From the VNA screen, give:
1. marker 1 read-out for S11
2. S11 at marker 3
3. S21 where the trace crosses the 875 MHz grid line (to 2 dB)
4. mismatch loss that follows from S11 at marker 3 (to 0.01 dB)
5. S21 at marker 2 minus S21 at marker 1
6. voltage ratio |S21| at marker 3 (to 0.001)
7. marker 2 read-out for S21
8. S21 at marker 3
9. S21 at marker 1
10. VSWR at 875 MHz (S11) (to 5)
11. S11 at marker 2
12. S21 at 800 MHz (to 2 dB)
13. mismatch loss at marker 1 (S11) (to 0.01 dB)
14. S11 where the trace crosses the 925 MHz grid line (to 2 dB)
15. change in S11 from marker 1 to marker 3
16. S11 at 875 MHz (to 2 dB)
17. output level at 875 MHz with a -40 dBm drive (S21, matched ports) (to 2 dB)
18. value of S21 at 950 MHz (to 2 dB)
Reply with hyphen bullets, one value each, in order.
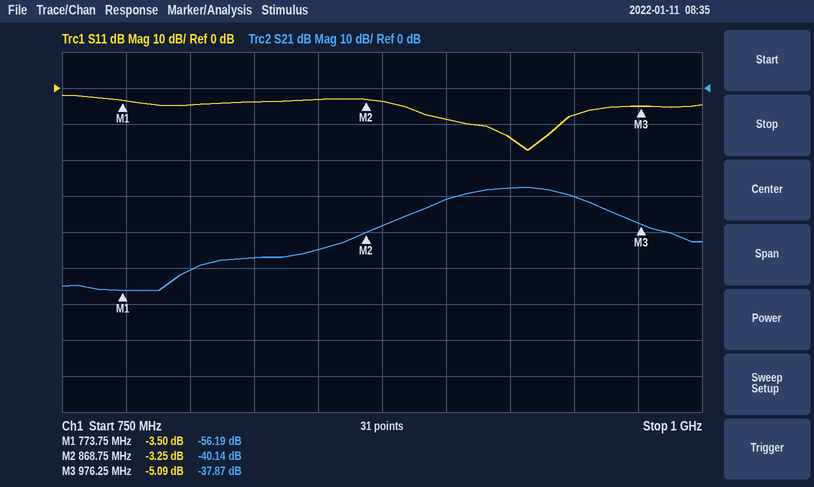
- -3.50 dB
- -5.09 dB
- -38 dB
- 1.61 dB
- 16.05 dB
- 0.013
- -40.14 dB
- -37.87 dB
- -56.19 dB
- 5
- -3.25 dB
- -50 dB
- 2.57 dB
- -14 dB
- -1.59 dB
- -4 dB
- -78 dBm
- -30 dB
